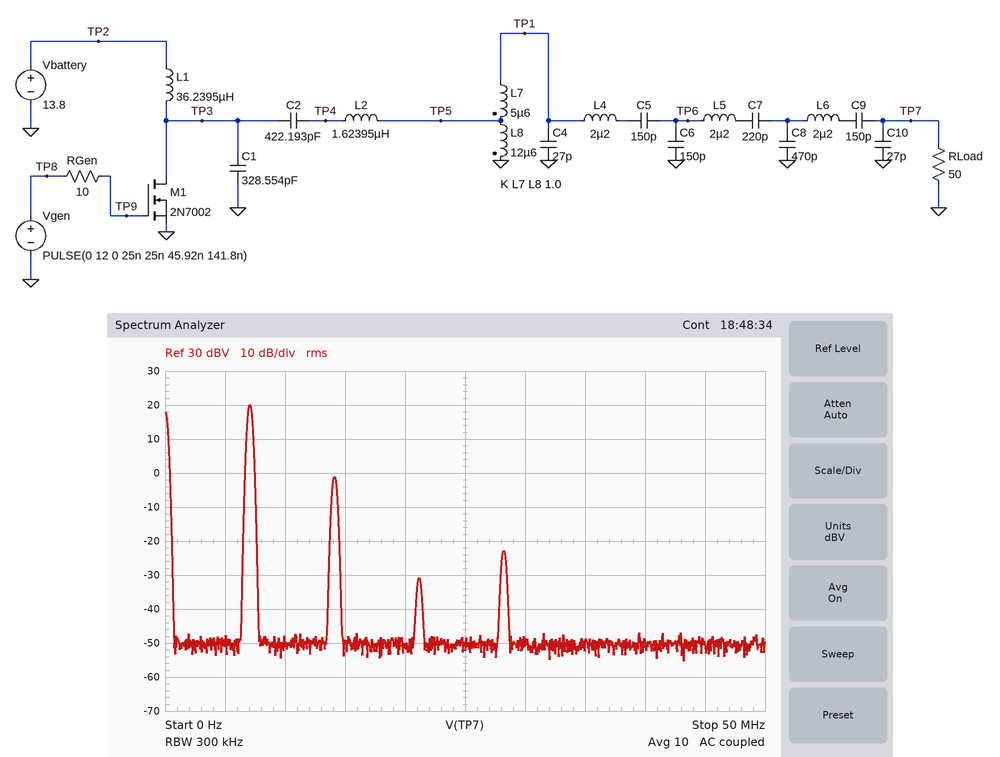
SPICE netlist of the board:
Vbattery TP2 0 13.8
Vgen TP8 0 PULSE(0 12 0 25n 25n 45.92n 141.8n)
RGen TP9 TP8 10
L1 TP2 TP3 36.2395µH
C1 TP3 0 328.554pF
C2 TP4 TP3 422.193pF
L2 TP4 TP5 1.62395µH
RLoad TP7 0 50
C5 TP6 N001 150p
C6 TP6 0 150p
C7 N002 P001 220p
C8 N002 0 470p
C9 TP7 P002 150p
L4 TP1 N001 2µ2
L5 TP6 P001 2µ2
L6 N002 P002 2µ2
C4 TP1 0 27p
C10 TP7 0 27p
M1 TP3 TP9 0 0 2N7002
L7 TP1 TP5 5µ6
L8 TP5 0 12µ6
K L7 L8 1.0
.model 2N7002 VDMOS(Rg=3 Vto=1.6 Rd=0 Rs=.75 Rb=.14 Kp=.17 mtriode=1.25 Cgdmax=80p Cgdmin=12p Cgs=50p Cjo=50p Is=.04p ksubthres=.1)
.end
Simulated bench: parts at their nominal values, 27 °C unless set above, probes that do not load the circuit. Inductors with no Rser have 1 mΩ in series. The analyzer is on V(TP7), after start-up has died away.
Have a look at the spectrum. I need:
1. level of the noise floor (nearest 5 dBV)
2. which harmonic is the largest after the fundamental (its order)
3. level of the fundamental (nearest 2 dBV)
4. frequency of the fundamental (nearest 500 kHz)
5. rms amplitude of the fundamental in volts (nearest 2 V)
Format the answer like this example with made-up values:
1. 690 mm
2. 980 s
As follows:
1. -50 dBV
2. 2
3. 20 dBV
4. 7.0 MHz
5. 10 V
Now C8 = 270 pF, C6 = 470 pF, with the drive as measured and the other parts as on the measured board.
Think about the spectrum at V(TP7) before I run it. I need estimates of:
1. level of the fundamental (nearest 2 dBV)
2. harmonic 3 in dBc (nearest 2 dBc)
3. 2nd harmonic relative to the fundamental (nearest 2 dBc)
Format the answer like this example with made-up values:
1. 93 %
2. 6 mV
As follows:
1. 20 dBV
2. -56 dBc
3. -30 dBc
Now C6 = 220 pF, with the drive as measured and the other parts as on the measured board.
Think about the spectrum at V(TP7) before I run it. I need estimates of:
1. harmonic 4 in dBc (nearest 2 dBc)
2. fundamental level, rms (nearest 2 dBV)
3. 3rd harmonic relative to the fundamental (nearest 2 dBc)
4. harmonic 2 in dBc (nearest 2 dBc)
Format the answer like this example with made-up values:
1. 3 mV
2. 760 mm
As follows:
1. -58 dBc
2. 20 dBV
3. -54 dBc
4. -28 dBc
